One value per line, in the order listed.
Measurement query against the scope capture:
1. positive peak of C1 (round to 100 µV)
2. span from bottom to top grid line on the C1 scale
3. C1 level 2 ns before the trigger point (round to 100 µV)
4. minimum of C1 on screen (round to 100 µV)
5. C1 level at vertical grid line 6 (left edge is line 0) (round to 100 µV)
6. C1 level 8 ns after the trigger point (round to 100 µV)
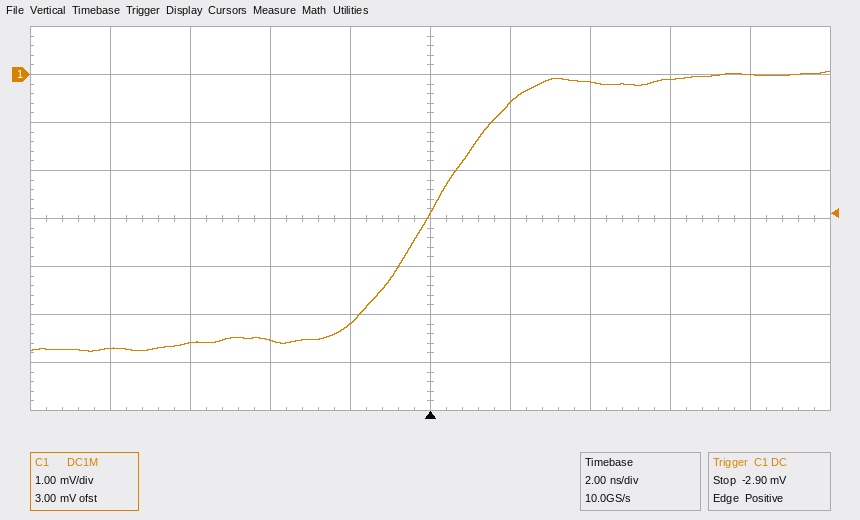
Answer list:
100 µV
8 mV
-5.2 mV
-5.8 mV
-600 µV
0.0 mV
